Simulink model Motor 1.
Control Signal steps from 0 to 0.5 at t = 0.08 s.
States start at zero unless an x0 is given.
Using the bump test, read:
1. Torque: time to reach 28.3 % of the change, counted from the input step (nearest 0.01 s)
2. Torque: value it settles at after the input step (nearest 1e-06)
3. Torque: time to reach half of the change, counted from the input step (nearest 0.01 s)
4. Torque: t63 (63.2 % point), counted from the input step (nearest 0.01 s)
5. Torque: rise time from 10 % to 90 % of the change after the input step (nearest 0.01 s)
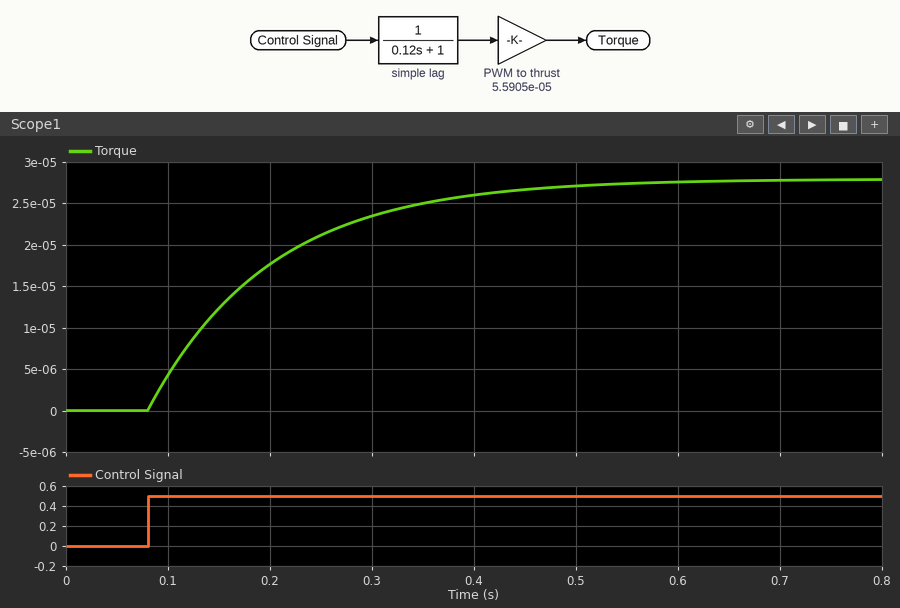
0.04 s
0.000028
0.08 s
0.12 s
0.26 s
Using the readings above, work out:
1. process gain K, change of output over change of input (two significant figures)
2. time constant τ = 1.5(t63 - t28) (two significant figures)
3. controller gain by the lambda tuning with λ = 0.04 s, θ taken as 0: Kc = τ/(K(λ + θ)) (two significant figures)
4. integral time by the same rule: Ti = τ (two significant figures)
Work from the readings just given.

0.000056
0.12 s
54000
0.12 s
